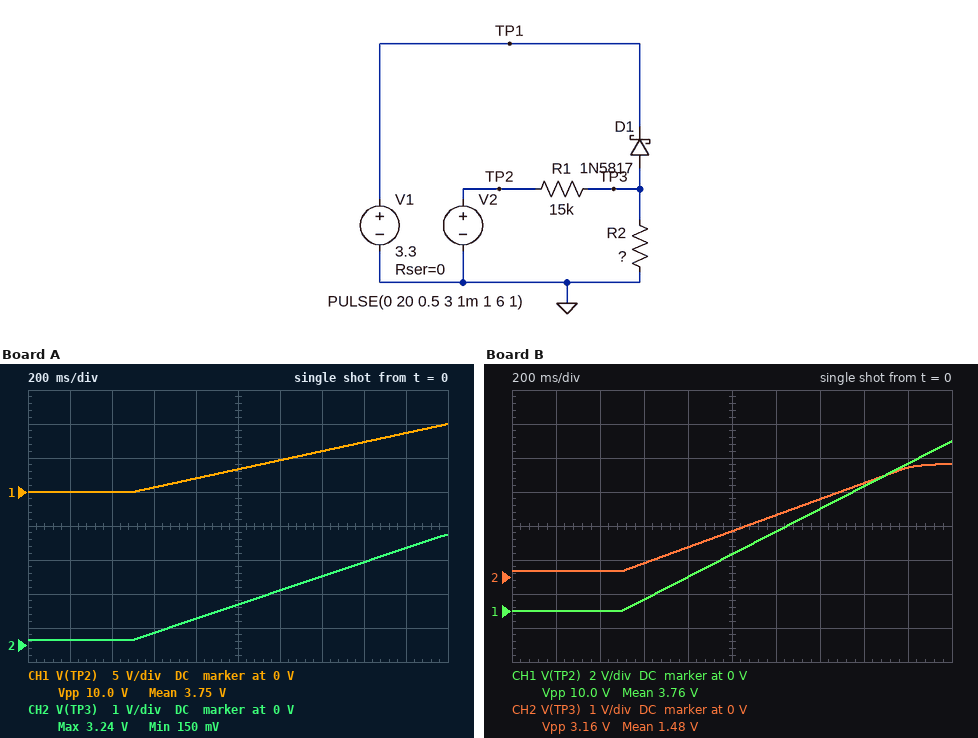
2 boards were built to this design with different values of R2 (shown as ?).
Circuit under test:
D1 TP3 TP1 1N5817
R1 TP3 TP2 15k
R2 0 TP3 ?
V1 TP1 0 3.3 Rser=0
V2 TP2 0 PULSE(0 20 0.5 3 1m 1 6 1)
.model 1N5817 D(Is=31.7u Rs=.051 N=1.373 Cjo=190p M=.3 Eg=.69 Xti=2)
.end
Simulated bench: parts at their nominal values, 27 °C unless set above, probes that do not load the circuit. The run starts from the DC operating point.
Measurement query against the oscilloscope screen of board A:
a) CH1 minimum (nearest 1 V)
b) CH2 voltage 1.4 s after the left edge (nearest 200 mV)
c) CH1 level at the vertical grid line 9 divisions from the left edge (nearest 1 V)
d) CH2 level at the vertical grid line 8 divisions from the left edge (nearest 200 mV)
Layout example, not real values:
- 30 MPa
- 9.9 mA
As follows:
- 0 V
- 2.0 V
- 9 V
- 2.4 V
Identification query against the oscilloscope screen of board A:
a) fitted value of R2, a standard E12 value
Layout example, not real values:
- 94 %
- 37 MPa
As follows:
- 6.8 kΩ
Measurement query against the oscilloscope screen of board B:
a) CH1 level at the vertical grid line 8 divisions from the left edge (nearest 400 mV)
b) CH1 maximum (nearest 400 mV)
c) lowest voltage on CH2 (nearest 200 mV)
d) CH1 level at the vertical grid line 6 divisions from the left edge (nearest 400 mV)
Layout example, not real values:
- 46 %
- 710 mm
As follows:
- 7.2 V
- 10.0 V
- 200 mV
- 4.8 V
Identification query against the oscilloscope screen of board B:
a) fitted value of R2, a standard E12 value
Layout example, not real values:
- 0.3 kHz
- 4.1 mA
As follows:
- 8.2 kΩ
